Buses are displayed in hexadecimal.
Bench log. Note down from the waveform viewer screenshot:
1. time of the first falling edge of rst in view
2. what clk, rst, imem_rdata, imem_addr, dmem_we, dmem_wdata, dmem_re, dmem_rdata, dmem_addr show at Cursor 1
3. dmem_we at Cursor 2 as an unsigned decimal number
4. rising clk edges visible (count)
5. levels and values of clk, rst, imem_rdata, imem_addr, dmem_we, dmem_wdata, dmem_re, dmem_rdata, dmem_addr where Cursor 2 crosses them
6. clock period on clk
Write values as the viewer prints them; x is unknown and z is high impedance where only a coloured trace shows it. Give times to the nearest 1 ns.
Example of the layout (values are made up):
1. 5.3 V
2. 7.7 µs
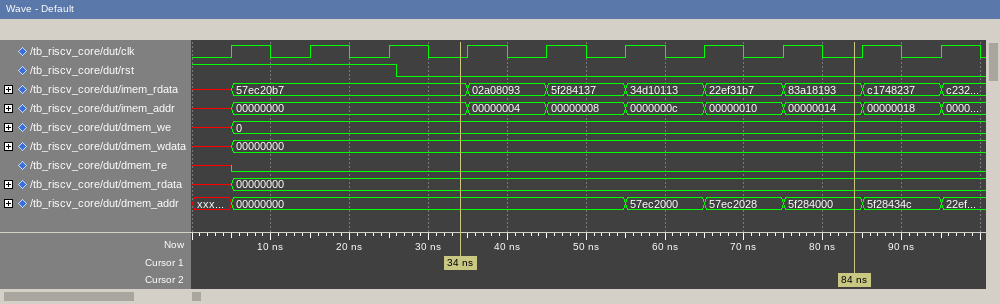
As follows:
1. 26 ns
2. clk=0, rst=0, imem_rdata=57ec20b7, imem_addr=00000000, dmem_we=0, dmem_wdata=00000000, dmem_re=0, dmem_rdata=00000000, dmem_addr=00000000
3. 0
4. 10
5. clk=0, rst=0, imem_rdata=83a18193, imem_addr=00000014, dmem_we=0, dmem_wdata=00000000, dmem_re=0, dmem_rdata=00000000, dmem_addr=5f284000
6. 10 ns
